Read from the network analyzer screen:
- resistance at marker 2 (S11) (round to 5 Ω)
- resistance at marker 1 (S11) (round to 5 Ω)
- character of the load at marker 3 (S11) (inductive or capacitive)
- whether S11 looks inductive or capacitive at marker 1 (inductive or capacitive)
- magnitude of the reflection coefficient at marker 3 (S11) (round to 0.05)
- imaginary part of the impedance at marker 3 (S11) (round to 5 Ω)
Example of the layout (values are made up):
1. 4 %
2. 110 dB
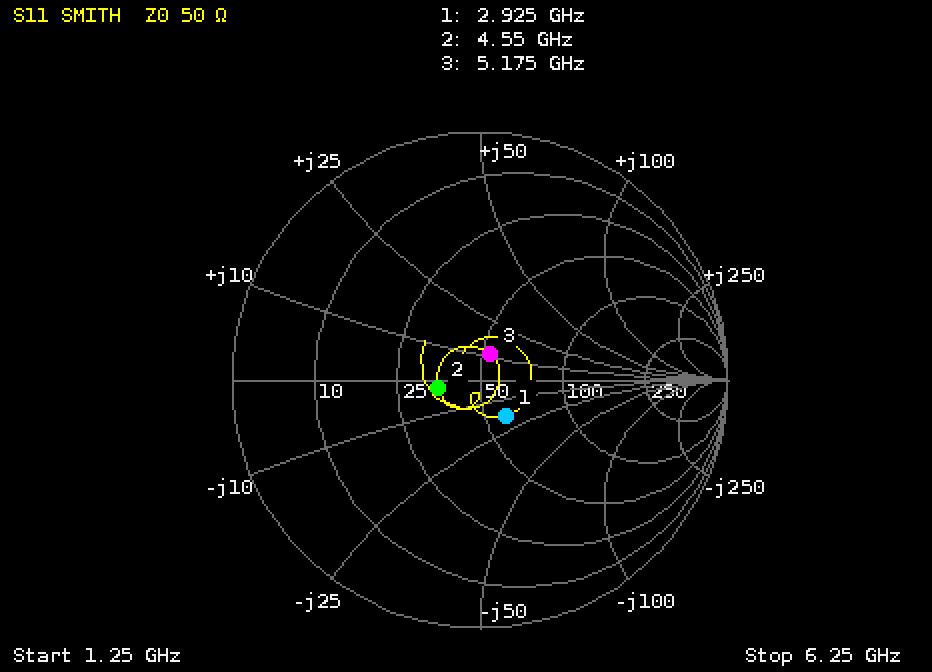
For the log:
1. 35 Ω
2. 60 Ω
3. inductive
4. capacitive
5. 0.10
6. +10 Ω
